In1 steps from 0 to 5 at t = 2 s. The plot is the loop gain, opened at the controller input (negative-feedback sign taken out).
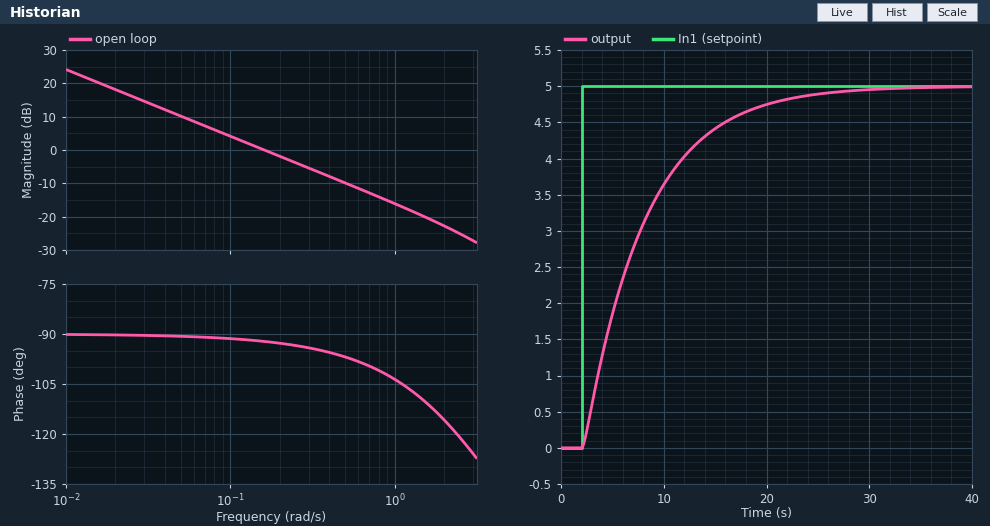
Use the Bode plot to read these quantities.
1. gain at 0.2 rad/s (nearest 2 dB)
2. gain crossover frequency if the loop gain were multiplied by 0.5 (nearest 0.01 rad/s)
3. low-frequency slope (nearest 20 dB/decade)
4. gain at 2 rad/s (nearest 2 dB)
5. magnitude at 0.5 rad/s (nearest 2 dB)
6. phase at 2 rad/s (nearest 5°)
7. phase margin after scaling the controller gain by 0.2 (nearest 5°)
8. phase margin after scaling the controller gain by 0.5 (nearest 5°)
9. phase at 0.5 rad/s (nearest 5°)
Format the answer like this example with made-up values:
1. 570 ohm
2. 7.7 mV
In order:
1. -2 dB
2. 0.08 rad/s
3. -20 dB/decade
4. -22 dB
5. -10 dB
6. -115°
7. 90°
8. 90°
9. -95°
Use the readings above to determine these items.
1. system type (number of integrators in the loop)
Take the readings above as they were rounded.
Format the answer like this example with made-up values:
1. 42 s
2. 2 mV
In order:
1. 1
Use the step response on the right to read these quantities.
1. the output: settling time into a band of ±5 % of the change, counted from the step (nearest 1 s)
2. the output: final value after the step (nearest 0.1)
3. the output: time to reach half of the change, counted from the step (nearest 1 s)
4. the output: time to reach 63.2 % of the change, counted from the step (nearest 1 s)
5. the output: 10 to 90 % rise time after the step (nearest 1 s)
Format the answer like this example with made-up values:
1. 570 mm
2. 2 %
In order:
1. 18 s
2. 5.0
3. 4 s
4. 6 s
5. 13 s
